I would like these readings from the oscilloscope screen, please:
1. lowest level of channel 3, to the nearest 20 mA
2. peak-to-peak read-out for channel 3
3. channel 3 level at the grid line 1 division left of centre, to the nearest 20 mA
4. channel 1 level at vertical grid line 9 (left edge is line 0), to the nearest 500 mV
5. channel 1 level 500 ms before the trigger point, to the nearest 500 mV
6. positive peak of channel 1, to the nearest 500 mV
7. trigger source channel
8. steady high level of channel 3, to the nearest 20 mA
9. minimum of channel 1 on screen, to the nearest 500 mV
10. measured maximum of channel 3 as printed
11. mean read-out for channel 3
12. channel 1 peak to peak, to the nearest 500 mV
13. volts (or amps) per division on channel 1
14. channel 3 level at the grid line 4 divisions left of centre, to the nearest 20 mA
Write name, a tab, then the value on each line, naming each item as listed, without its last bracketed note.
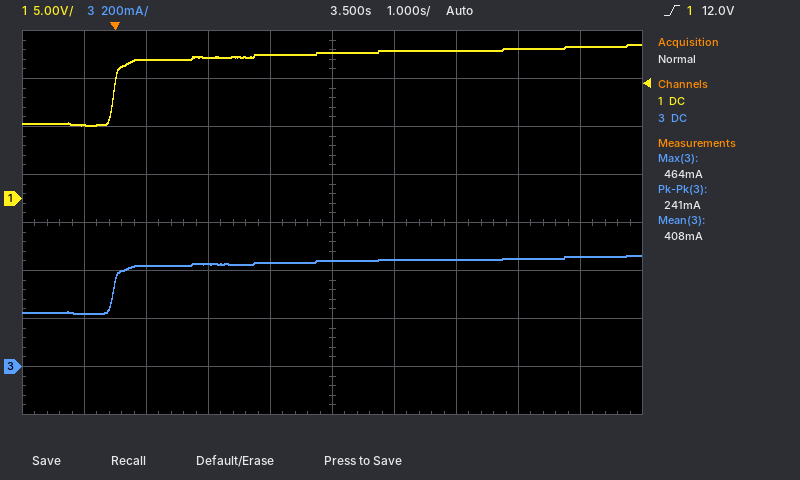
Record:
lowest level of channel 3, to the nearest 20 mA	220 mA
peak-to-peak read-out for channel 3	241 mA
channel 3 level at the grid line 1 division left of centre, to the nearest 20 mA	440 mA
channel 1 level at vertical grid line 9 (left edge is line 0), to the nearest 500 mV	16.0 V
channel 1 level 500 ms before the trigger point, to the nearest 500 mV	7.5 V
positive peak of channel 1, to the nearest 500 mV	16.0 V
trigger source channel	channel 1
steady high level of channel 3, to the nearest 20 mA	440 mA
minimum of channel 1 on screen, to the nearest 500 mV	7.5 V
measured maximum of channel 3 as printed	464 mA
mean read-out for channel 3	408 mA
channel 1 peak to peak, to the nearest 500 mV	8.5 V
volts (or amps) per division on channel 1	5 V
channel 3 level at the grid line 4 divisions left of centre, to the nearest 20 mA	220 mA
